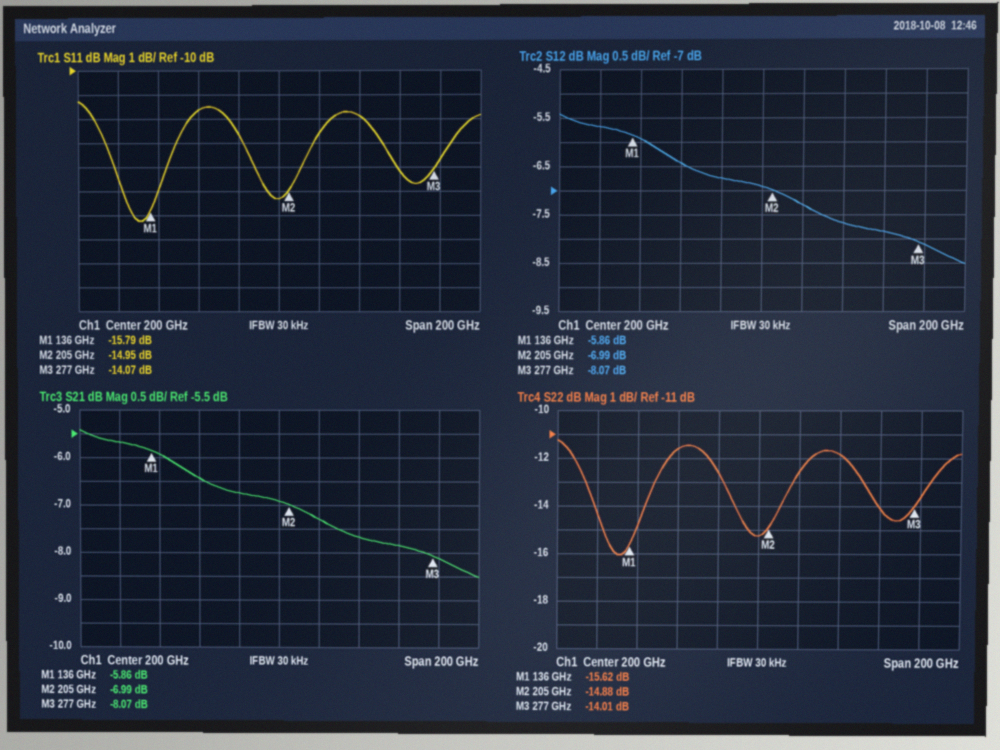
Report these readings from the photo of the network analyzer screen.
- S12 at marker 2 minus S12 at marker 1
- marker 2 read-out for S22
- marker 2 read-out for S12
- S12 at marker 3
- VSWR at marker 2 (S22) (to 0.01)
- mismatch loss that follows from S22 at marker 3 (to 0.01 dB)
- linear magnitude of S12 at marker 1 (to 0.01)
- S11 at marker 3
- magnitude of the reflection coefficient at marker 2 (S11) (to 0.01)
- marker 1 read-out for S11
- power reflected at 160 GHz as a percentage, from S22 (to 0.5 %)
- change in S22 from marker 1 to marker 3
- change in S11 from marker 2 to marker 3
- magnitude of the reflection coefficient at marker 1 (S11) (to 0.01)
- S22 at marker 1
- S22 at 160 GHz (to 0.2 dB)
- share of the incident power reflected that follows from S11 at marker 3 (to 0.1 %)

-1.13 dB
-14.88 dB
-6.99 dB
-8.07 dB
1.44
0.18 dB
0.51
-14.07 dB
0.18
-15.79 dB
7.0 %
1.61 dB
0.88 dB
0.16
-15.62 dB
-11.6 dB
3.9 %
